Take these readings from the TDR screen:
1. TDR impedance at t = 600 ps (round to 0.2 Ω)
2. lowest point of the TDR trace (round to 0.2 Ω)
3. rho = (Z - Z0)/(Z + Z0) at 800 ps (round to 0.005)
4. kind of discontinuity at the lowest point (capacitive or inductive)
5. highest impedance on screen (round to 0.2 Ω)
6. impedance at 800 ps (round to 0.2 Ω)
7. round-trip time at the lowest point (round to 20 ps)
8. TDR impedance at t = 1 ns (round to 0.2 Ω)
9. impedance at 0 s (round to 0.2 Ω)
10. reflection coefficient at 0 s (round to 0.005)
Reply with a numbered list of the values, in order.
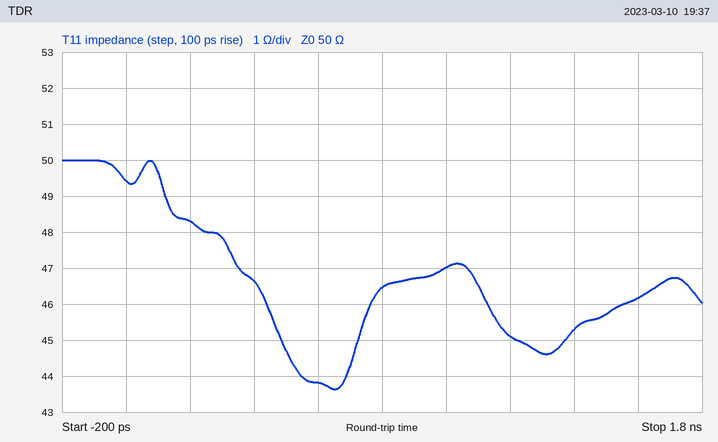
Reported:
1. 43.8 Ω
2. 43.6 Ω
3. -0.035
4. capacitive
5. 50.0 Ω
6. 46.4 Ω
7. 660 ps
8. 47.0 Ω
9. 49.4 Ω
10. -0.005
